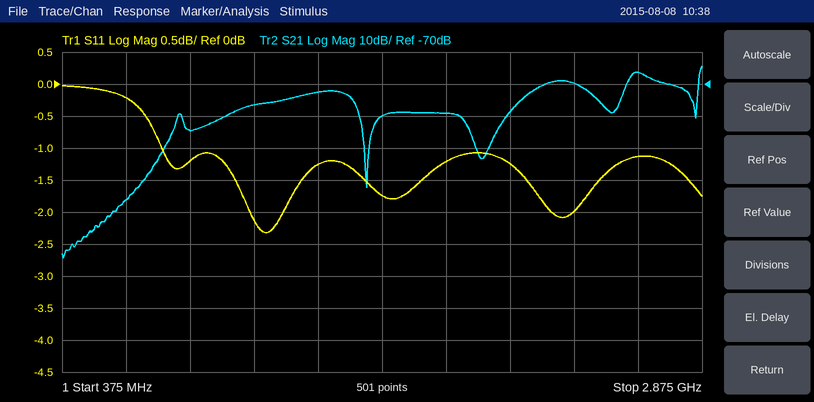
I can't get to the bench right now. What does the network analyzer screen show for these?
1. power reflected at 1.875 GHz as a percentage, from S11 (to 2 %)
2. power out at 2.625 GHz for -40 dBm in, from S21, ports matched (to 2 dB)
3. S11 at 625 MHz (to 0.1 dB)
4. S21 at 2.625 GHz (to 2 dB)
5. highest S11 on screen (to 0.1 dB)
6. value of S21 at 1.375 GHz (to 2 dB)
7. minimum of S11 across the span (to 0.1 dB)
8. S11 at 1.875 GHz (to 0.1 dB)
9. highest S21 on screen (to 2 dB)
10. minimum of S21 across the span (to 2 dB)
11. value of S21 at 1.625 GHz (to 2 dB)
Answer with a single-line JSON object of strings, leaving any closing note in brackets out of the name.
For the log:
{"power reflected at 1.875 GHz as a percentage, from S11": "76 %", "power out at 2.625 GHz for -40 dBm in, from S21, ports matched": "-106 dBm", "S11 at 625 MHz": "-0.2 dB", "S21 at 2.625 GHz": "-66 dB", "highest S11 on screen": "0.0 dB", "value of S21 at 1.375 GHz": "-72 dB", "minimum of S11 across the span": "-2.3 dB", "S11 at 1.875 GHz": "-1.2 dB", "highest S21 on screen": "-64 dB", "minimum of S21 across the span": "-124 dB", "value of S21 at 1.625 GHz": "-80 dB"}
